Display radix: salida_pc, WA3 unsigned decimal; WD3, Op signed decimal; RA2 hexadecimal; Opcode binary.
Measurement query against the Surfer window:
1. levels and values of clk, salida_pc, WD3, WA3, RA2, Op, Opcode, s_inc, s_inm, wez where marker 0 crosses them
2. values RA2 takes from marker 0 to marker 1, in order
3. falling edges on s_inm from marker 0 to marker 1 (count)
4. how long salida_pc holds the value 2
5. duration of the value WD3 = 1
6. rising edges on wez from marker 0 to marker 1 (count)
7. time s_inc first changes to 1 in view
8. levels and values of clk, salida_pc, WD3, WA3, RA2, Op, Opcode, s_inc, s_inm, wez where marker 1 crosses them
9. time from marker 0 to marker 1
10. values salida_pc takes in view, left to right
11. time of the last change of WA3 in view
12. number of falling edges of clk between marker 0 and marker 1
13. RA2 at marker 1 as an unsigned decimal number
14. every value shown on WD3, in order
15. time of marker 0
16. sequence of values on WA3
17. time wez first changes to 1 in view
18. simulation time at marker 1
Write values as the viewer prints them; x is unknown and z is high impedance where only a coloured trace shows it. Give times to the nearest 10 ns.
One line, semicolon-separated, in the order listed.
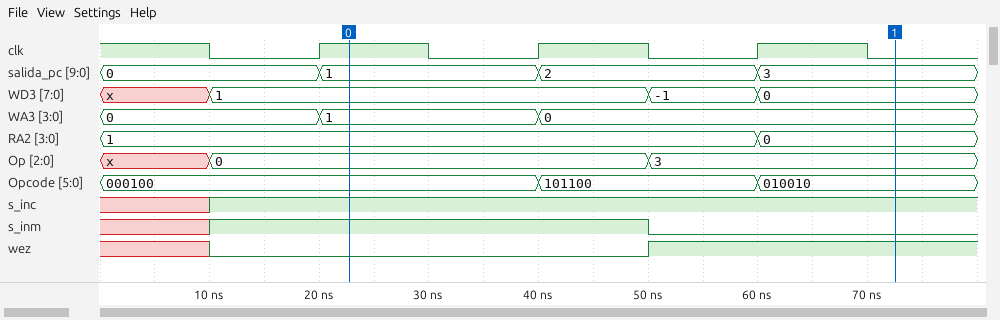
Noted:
clk=1, salida_pc=1, WD3=1, WA3=1, RA2=1, Op=0, Opcode=000100, s_inc=1, s_inm=1, wez=0; 1, 0; 1; 20 ns; 40 ns; 1; 10 ns; clk=0, salida_pc=3, WD3=0, WA3=0, RA2=0, Op=3, Opcode=010010, s_inc=1, s_inm=0, wez=1; 50 ns; 0, 1, 2, 3; 40 ns; 3; 0; x, 1, -1, 0; 20 ns; 0, 1, 0; 50 ns; 70 ns
